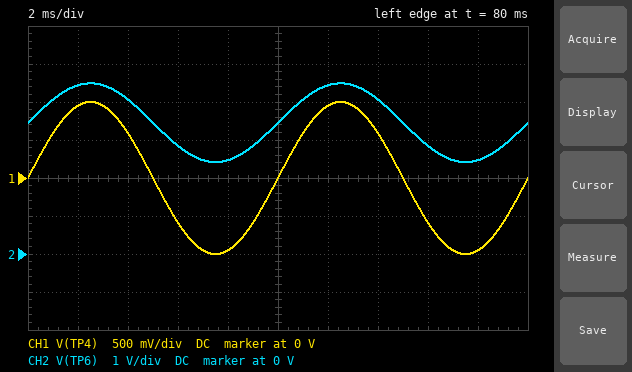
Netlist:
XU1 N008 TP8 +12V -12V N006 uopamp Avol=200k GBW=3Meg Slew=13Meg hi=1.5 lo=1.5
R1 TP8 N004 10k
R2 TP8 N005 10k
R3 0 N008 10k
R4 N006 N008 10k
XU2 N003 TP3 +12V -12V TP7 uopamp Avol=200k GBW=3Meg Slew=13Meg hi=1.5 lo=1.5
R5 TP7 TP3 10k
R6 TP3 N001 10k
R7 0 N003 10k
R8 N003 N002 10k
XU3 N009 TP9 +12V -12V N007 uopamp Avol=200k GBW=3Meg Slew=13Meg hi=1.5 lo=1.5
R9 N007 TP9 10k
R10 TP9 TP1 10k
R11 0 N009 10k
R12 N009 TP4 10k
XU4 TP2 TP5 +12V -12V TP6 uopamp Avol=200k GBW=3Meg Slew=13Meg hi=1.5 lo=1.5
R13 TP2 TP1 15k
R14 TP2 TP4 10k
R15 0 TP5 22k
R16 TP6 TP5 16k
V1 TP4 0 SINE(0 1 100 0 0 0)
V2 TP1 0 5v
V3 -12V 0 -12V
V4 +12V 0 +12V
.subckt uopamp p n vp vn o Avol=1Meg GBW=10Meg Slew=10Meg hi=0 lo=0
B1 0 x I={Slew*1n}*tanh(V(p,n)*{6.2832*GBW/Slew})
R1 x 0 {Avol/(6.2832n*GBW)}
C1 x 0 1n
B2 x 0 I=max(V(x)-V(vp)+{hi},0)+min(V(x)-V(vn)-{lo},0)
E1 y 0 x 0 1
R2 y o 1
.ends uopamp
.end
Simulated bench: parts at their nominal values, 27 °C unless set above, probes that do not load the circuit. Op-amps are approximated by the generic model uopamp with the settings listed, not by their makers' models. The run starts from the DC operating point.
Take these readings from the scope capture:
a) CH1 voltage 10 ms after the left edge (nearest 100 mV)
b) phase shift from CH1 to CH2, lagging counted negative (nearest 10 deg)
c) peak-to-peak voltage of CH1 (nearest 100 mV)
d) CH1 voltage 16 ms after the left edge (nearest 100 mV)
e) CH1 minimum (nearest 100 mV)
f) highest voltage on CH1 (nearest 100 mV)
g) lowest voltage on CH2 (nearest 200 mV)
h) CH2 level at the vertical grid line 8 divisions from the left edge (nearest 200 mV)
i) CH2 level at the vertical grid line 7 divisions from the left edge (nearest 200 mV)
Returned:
0 V
0 deg
2.0 V
-600 mV
-1.0 V
1.0 V
2.4 V
2.8 V
4.0 V
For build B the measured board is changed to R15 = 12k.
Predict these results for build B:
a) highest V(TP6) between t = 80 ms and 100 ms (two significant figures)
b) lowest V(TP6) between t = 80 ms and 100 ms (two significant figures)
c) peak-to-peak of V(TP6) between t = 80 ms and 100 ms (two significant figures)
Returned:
6.1 V
3.3 V
2.8 V
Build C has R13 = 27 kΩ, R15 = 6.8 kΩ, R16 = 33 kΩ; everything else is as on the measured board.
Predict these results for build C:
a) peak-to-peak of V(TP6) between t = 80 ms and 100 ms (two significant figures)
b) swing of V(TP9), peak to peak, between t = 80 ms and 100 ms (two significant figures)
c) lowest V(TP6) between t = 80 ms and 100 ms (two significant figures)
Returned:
6.9 V
1.0 V
3.6 V
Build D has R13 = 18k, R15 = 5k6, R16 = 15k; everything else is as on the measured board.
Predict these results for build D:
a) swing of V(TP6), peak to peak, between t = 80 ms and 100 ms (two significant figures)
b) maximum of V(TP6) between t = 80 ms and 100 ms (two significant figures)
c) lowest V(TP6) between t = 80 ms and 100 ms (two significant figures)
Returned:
4.7 V
8.9 V
4.2 V
